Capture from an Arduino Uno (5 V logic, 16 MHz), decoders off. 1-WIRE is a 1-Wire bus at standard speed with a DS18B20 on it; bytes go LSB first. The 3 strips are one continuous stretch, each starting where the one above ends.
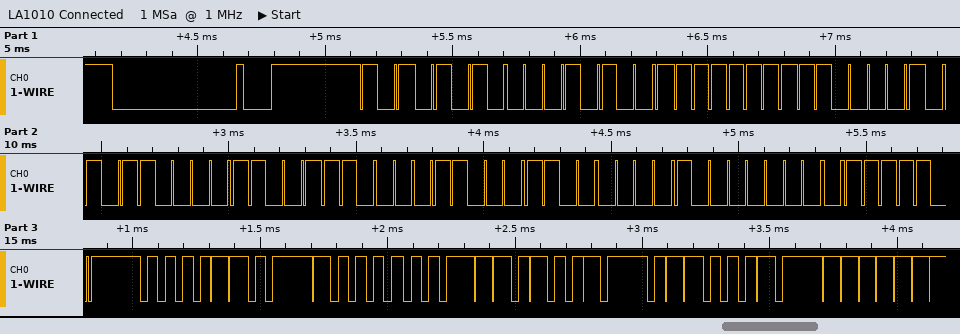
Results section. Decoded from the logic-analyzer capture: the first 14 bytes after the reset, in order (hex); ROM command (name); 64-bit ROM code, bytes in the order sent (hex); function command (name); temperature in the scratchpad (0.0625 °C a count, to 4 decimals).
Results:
55 28 FF 43 0D 73 18 03 01 BE 30 01 4B 46
Match ROM
28 FF 43 0D 73 18 03 01
Read Scratchpad
19.0000 °C
